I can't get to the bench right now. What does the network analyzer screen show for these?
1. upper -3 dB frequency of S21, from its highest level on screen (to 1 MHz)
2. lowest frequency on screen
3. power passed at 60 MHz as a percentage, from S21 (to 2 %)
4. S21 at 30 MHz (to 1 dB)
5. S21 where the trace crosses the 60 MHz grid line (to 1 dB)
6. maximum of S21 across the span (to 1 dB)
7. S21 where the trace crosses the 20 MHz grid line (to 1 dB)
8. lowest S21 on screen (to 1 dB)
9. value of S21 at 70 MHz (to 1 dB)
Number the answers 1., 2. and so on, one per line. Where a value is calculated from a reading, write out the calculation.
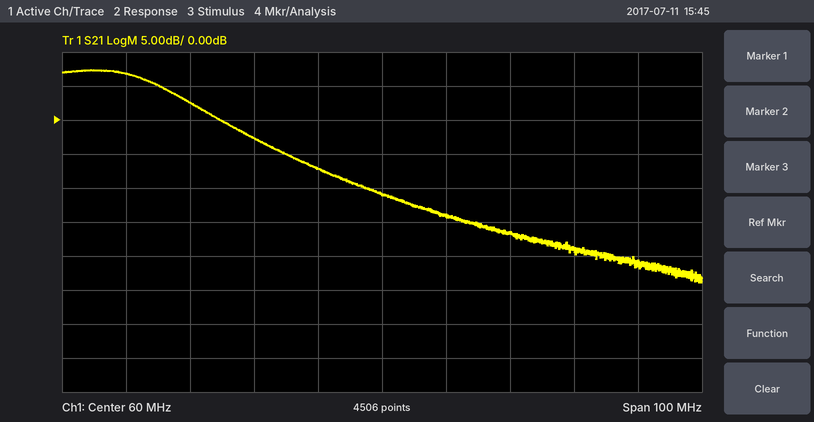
1. 26 MHz
2. 10 MHz
3. 10^(-11/10) ≈ 8 %
4. 3 dB
5. -11 dB
6. 7 dB
7. 7 dB
8. -24 dB
9. -14 dB
